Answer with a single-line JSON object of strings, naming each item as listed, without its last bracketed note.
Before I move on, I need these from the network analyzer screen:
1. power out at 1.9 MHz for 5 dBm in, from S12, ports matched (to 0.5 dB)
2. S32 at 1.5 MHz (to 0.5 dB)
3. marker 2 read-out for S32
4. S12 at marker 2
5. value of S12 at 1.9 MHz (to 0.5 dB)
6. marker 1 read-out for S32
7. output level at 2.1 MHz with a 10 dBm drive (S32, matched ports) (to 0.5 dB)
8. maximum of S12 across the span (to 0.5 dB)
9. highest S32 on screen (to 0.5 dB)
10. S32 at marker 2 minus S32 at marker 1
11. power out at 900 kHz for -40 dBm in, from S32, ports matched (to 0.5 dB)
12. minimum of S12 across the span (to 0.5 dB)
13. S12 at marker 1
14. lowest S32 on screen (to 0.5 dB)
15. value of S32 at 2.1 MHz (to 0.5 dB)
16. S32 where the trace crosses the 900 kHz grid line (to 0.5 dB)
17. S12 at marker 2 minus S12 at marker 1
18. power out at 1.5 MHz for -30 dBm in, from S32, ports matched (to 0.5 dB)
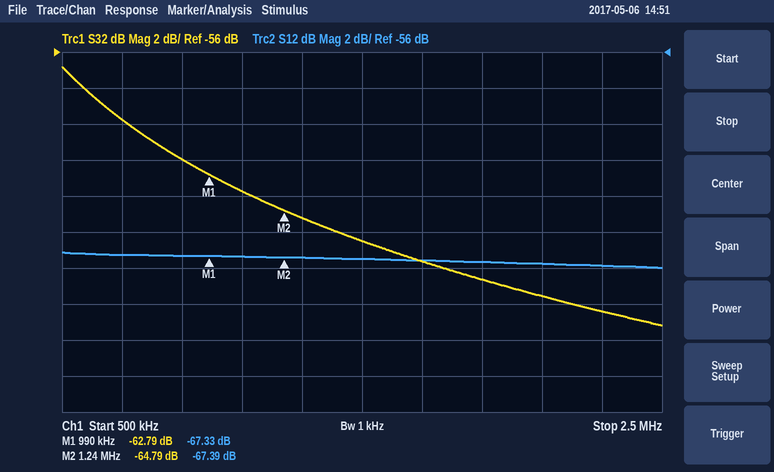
{"power out at 1.9 MHz for 5 dBm in, from S12, ports matched": "-62.5 dBm", "S32 at 1.5 MHz": "-66.5 dB", "marker 2 read-out for S32": "-64.79 dB", "S12 at marker 2": "-67.39 dB", "value of S12 at 1.9 MHz": "-67.5 dB", "marker 1 read-out for S32": "-62.79 dB", "output level at 2.1 MHz with a 10 dBm drive (S32, matched ports)": "-59.5 dBm", "maximum of S12 across the span": "-67.0 dB", "highest S32 on screen": "-57.0 dB", "S32 at marker 2 minus S32 at marker 1": "-2.00 dB", "power out at 900 kHz for -40 dBm in, from S32, ports matched": "-102.0 dBm", "minimum of S12 across the span": "-68.0 dB", "S12 at marker 1": "-67.33 dB", "lowest S32 on screen": "-71.0 dB", "value of S32 at 2.1 MHz": "-69.5 dB", "S32 where the trace crosses the 900 kHz grid line": "-62.0 dB", "S12 at marker 2 minus S12 at marker 1": "-0.06 dB", "power out at 1.5 MHz for -30 dBm in, from S32, ports matched": "-96.5 dBm"}
